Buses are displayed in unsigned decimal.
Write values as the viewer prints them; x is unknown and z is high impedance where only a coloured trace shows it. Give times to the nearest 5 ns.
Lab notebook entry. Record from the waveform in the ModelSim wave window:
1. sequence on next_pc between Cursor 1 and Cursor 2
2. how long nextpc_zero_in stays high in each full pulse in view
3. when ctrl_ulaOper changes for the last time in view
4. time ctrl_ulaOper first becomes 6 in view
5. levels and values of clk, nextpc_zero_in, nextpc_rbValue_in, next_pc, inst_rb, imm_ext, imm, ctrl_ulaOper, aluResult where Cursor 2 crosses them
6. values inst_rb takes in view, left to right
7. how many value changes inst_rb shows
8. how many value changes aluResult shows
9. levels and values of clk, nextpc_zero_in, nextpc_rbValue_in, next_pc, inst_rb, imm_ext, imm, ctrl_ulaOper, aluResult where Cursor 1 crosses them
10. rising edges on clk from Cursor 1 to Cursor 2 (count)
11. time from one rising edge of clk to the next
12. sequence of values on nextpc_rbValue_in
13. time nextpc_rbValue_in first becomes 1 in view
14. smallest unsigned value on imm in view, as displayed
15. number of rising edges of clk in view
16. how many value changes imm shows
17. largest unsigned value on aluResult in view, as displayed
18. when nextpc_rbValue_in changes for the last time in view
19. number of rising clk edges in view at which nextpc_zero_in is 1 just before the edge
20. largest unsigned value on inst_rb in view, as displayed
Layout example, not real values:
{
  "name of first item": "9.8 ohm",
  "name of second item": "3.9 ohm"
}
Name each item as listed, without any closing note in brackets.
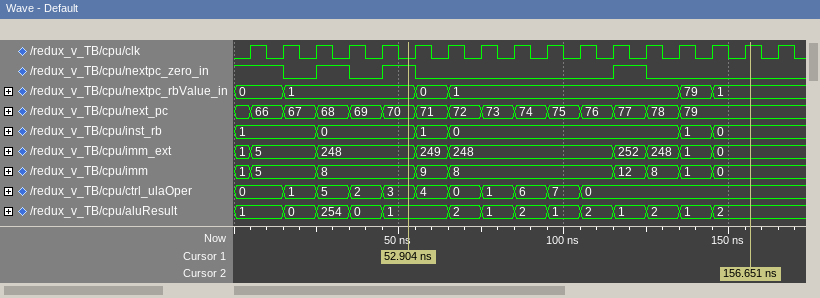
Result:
{
  "sequence on next_pc between Cursor 1 and Cursor 2": "70, 71, 72, 73, 74, 75, 76, 77, 78, 79",
  "how long nextpc_zero_in stays high in each full pulse in view": "10 ns, 10 ns, 10 ns",
  "when ctrl_ulaOper changes for the last time in view": "105 ns",
  "time ctrl_ulaOper first becomes 6 in view": "85 ns",
  "levels and values of clk, nextpc_zero_in, nextpc_rbValue_in, next_pc, inst_rb, imm_ext, imm, ctrl_ulaOper, aluResult where Cursor 2 crosses them": "clk=1, nextpc_zero_in=0, nextpc_rbValue_in=1, next_pc=79, inst_rb=0, imm_ext=0, imm=0, ctrl_ulaOper=0, aluResult=2",
  "values inst_rb takes in view, left to right": "1, 0, 1, 0, 1, 0",
  "how many value changes inst_rb shows": "5",
  "how many value changes aluResult shows": "13",
  "levels and values of clk, nextpc_zero_in, nextpc_rbValue_in, next_pc, inst_rb, imm_ext, imm, ctrl_ulaOper, aluResult where Cursor 1 crosses them": "clk=0, nextpc_zero_in=1, nextpc_rbValue_in=1, next_pc=70, inst_rb=0, imm_ext=248, imm=8, ctrl_ulaOper=3, aluResult=1",
  "rising edges on clk from Cursor 1 to Cursor 2": "11",
  "time from one rising edge of clk to the next": "10 ns",
  "sequence of values on nextpc_rbValue_in": "0, 1, 0, 1, 79, 1",
  "time nextpc_rbValue_in first becomes 1 in view": "15 ns",
  "smallest unsigned value on imm in view, as displayed": "0",
  "number of rising edges of clk in view": "17",
  "how many value changes imm shows": "8",
  "largest unsigned value on aluResult in view, as displayed": "254",
  "when nextpc_rbValue_in changes for the last time in view": "145 ns",
  "number of rising clk edges in view at which nextpc_zero_in is 1 just before the edge": "5",
  "largest unsigned value on inst_rb in view, as displayed": "1"
}
